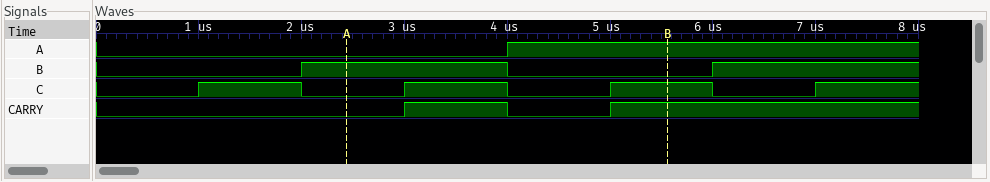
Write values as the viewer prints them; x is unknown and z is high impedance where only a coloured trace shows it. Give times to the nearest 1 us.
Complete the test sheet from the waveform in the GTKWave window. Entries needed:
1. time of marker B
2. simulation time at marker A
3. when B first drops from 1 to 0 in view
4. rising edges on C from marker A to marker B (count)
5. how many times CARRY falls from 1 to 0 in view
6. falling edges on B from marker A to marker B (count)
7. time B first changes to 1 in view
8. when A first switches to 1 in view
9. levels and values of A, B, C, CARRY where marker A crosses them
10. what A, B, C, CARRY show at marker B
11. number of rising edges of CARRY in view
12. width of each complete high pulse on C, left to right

6 us
2 us
4 us
2
1
1
2 us
4 us
A=0, B=1, C=0, CARRY=0
A=1, B=0, C=1, CARRY=1
2
1 us, 1 us, 1 us
